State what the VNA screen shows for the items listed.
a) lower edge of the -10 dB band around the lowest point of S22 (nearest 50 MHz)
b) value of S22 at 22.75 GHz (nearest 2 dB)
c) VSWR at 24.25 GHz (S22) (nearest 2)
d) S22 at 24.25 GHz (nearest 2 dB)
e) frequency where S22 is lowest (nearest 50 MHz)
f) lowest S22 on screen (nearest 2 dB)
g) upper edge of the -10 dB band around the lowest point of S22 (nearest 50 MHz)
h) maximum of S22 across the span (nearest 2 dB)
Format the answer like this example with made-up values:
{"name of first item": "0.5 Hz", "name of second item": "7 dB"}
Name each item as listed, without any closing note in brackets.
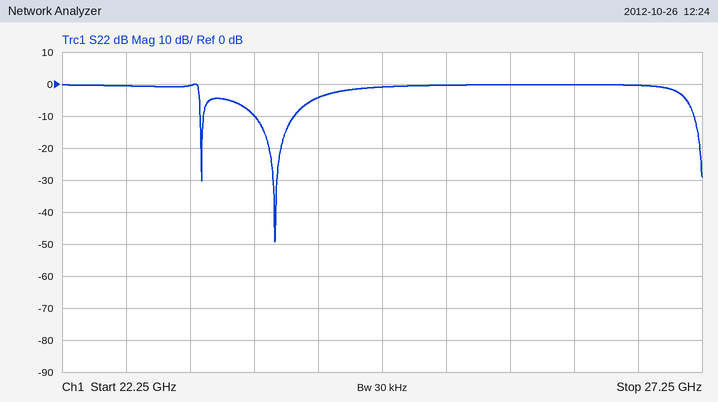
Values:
{"lower edge of the -10 dB band around the lowest point of S22": "23.75 GHz", "value of S22 at 22.75 GHz": "0 dB", "VSWR at 24.25 GHz (S22)": "4", "S22 at 24.25 GHz": "-4 dB", "frequency where S22 is lowest": "23.90 GHz", "lowest S22 on screen": "-50 dB", "upper edge of the -10 dB band around the lowest point of S22": "24.05 GHz", "maximum of S22 across the span": "0 dB"}
